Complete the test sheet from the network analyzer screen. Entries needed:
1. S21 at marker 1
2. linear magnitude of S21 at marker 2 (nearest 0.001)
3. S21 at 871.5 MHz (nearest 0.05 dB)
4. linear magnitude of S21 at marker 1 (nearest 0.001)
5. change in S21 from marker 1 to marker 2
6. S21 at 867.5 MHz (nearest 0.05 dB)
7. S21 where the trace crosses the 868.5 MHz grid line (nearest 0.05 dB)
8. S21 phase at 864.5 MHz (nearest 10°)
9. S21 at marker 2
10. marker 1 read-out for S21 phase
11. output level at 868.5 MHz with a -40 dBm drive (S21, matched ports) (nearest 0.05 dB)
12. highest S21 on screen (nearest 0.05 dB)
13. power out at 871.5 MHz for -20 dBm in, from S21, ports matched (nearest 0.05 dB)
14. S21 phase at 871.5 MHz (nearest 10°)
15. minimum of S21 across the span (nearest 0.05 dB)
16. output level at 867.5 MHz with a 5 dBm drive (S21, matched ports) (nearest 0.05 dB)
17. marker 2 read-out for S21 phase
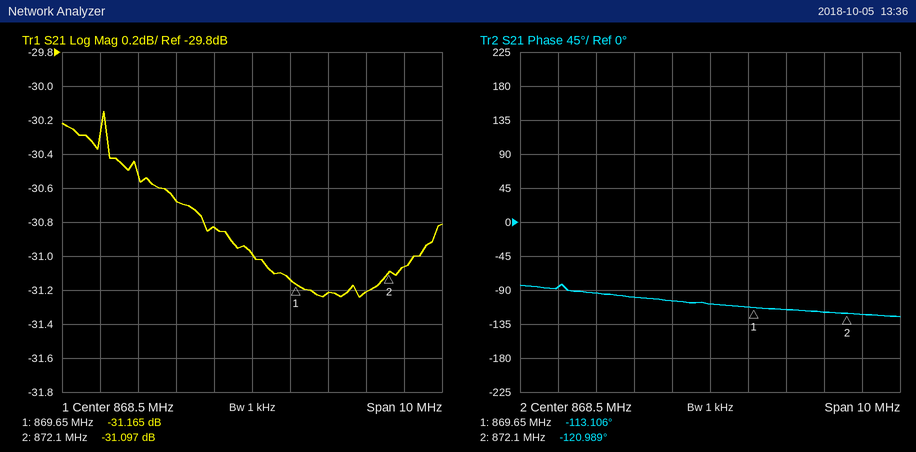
-31.165 dB
0.028
-31.20 dB
0.028
0.068 dB
-30.85 dB
-31.00 dB
-90°
-31.097 dB
-113.106°
-71.00 dBm
-30.15 dB
-51.20 dBm
-120°
-31.25 dB
-25.85 dBm
-120.989°
